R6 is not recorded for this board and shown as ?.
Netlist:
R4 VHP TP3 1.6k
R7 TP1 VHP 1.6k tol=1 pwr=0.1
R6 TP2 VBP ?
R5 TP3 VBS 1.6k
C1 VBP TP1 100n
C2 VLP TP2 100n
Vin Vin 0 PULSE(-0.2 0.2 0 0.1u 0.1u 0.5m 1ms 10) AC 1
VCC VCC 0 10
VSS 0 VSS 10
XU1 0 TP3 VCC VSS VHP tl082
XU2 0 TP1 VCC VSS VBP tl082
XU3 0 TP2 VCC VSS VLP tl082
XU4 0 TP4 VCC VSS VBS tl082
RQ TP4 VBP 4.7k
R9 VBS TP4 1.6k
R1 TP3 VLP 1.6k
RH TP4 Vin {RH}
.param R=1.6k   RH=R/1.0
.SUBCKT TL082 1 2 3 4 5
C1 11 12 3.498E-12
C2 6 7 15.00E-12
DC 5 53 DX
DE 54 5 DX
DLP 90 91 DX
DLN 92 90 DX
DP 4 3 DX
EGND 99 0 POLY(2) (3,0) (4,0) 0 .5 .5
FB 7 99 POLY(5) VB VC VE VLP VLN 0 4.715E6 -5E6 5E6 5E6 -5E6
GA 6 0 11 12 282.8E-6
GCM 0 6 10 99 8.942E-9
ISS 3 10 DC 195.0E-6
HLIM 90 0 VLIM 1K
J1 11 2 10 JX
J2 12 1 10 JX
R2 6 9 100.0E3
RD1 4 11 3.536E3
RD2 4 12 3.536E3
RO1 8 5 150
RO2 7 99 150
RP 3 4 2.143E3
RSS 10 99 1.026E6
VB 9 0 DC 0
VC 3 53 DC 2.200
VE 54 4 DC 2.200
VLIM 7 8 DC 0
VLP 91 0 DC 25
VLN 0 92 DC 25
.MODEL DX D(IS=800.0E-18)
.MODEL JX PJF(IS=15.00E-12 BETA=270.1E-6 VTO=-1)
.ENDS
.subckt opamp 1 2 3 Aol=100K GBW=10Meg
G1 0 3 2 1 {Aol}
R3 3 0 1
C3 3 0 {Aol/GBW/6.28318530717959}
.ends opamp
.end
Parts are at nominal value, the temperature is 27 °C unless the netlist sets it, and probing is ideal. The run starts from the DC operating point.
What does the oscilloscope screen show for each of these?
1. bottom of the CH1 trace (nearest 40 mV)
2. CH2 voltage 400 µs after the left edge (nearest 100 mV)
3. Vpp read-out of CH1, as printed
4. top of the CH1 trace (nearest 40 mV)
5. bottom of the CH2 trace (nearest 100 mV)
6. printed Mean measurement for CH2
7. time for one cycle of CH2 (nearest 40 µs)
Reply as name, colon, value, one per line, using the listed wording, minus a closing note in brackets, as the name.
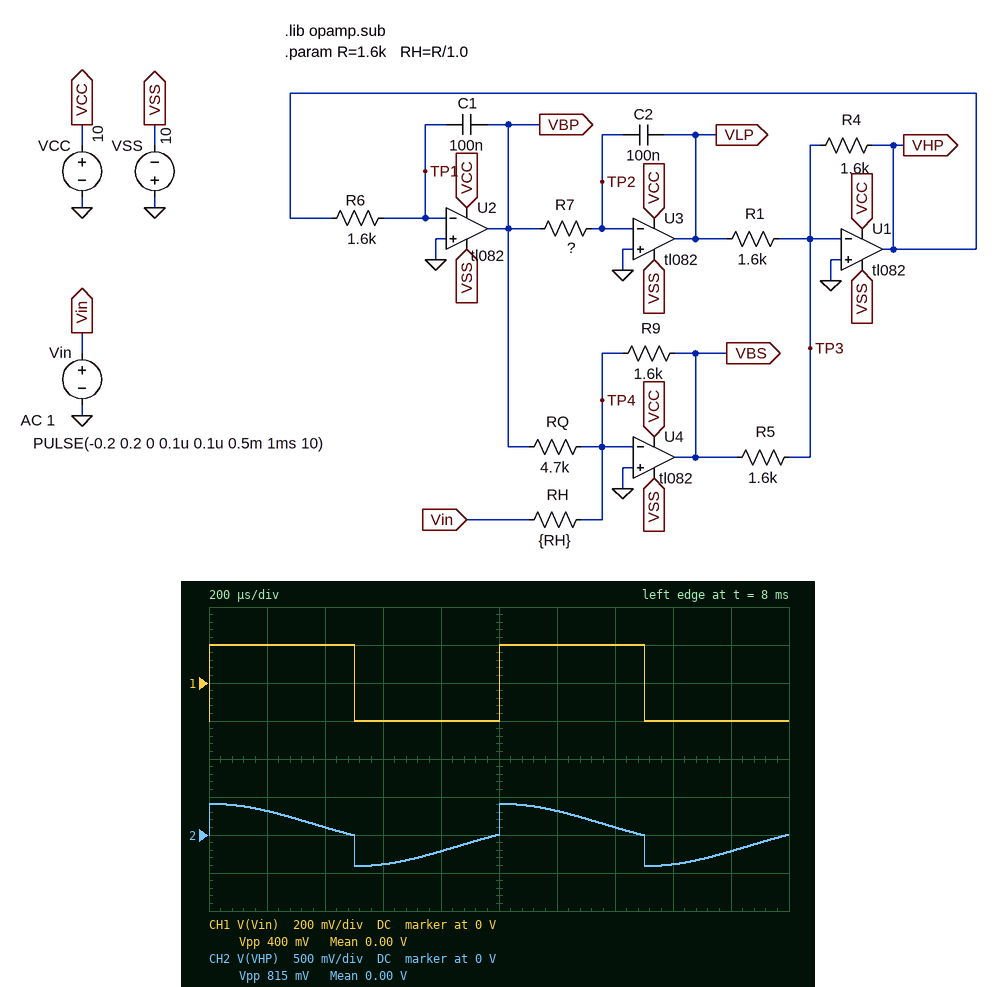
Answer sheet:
bottom of the CH1 trace: -200 mV
CH2 voltage 400 µs after the left edge: 100 mV
Vpp read-out of CH1, as printed: 400 mV
top of the CH1 trace: 200 mV
bottom of the CH2 trace: -400 mV
printed Mean measurement for CH2: 0.00 V
time for one cycle of CH2: 1.00 ms
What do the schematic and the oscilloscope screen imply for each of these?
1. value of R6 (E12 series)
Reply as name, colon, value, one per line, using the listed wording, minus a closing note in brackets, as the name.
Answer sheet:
value of R6: 3.9 kΩ
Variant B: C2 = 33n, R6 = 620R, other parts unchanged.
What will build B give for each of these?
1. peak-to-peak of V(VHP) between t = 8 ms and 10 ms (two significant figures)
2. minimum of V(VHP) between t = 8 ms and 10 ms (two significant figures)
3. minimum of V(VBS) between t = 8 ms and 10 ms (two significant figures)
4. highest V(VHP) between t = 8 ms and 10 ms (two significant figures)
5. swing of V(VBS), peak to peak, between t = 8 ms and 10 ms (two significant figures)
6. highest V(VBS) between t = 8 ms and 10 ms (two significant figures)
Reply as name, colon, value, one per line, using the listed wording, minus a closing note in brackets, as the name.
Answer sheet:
peak-to-peak of V(VHP) between t = 8 ms and 10 ms: 1.2 V
minimum of V(VHP) between t = 8 ms and 10 ms: -580 mV
minimum of V(VBS) between t = 8 ms and 10 ms: -250 mV
highest V(VHP) between t = 8 ms and 10 ms: 580 mV
swing of V(VBS), peak to peak, between t = 8 ms and 10 ms: 510 mV
highest V(VBS) between t = 8 ms and 10 ms: 250 mV
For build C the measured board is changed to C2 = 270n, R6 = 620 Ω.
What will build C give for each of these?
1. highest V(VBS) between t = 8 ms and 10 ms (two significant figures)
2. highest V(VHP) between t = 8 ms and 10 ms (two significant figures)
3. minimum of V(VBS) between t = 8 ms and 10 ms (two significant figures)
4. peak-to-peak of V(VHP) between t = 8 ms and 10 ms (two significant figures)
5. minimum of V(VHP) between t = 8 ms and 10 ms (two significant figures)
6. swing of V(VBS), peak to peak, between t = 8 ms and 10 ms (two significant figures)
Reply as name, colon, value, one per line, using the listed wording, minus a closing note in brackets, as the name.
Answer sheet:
highest V(VBS) between t = 8 ms and 10 ms: 260 mV
highest V(VHP) between t = 8 ms and 10 ms: 960 mV
minimum of V(VBS) between t = 8 ms and 10 ms: -260 mV
peak-to-peak of V(VHP) between t = 8 ms and 10 ms: 1.9 V
minimum of V(VHP) between t = 8 ms and 10 ms: -960 mV
swing of V(VBS), peak to peak, between t = 8 ms and 10 ms: 520 mV
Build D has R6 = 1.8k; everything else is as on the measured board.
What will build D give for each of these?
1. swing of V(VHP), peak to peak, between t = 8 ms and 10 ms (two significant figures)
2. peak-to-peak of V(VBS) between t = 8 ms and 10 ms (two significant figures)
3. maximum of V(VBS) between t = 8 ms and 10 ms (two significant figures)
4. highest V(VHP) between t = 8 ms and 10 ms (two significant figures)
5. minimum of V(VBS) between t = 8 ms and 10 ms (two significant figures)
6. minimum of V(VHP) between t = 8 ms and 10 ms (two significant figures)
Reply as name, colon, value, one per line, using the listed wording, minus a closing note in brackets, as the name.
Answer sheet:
swing of V(VHP), peak to peak, between t = 8 ms and 10 ms: 1.8 V
peak-to-peak of V(VBS) between t = 8 ms and 10 ms: 600 mV
maximum of V(VBS) between t = 8 ms and 10 ms: 300 mV
highest V(VHP) between t = 8 ms and 10 ms: 890 mV
minimum of V(VBS) between t = 8 ms and 10 ms: -300 mV
minimum of V(VHP) between t = 8 ms and 10 ms: -890 mV
